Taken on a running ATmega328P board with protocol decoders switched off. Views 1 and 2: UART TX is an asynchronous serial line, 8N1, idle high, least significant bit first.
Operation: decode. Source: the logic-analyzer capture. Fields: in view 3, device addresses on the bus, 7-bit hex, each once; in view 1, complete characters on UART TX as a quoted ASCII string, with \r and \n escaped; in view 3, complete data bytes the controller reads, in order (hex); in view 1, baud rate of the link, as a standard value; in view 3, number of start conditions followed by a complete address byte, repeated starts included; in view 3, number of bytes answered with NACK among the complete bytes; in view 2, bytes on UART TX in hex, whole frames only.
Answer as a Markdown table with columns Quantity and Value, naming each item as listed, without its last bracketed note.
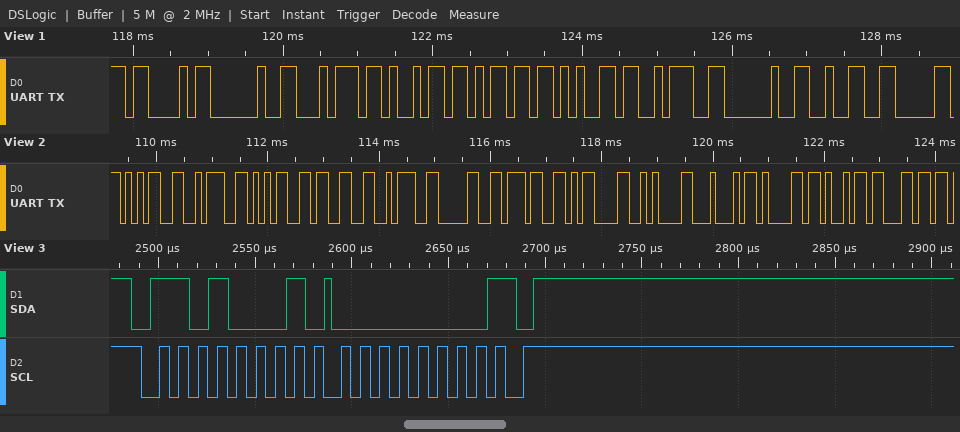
| Quantity | Value |
|---|---|
| in view 3, device addresses on the bus, 7-bit hex, each once | 0x68 |
| in view 1, complete characters on UART TX as a quoted ASCII string, with \r and \n escaped | "C time: 2" |
| in view 3, complete data bytes the controller reads, in order | 00 |
| in view 1, baud rate of the link, as a standard value | 9600 baud |
| in view 3, number of start conditions followed by a complete address byte, repeated starts included | 1 |
| in view 3, number of bytes answered with NACK among the complete bytes | 1 |
| in view 2, bytes on UART TX in hex, whole frames only | 35 3A 35 33 3A 30 37 0D 0A 44 61 69 6C |
